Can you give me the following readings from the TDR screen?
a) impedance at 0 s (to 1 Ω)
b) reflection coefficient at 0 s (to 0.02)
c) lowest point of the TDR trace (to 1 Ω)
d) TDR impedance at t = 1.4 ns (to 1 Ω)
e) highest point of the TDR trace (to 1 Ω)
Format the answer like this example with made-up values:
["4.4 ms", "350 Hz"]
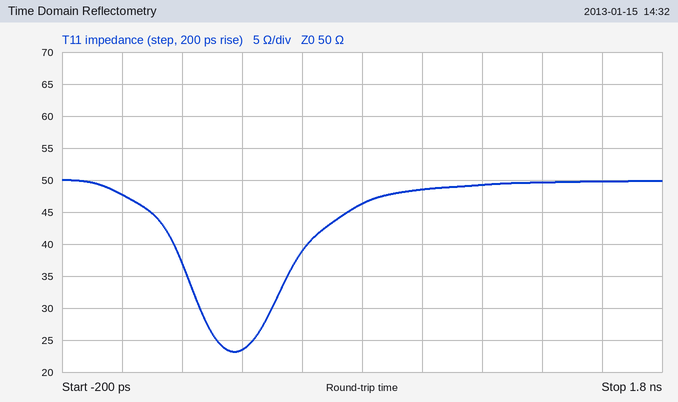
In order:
["48 Ω", "-0.02", "23 Ω", "50 Ω", "50 Ω"]
